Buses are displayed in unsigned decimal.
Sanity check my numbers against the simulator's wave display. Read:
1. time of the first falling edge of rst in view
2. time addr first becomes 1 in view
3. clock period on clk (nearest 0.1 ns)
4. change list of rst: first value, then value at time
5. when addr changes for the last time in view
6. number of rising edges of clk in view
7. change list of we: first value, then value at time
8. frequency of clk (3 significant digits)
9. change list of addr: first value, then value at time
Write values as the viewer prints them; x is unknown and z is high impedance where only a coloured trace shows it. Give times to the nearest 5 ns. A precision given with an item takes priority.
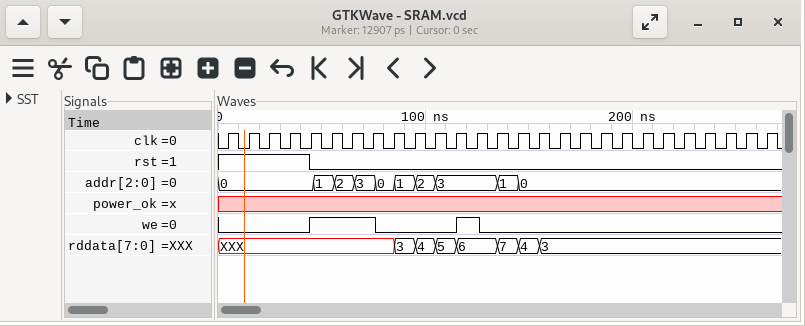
45 ns
45 ns
10 ns
1, 0 at 45 ns
145 ns
27
0, 1 at 45 ns, 0 at 75 ns, 1 at 115 ns, 0 at 125 ns
100 MHz
0, 1 at 45 ns, 2 at 55 ns, 3 at 65 ns, 0 at 75 ns, 1 at 85 ns, 2 at 95 ns, 3 at 105 ns, 1 at 135 ns, 0 at 145 ns
